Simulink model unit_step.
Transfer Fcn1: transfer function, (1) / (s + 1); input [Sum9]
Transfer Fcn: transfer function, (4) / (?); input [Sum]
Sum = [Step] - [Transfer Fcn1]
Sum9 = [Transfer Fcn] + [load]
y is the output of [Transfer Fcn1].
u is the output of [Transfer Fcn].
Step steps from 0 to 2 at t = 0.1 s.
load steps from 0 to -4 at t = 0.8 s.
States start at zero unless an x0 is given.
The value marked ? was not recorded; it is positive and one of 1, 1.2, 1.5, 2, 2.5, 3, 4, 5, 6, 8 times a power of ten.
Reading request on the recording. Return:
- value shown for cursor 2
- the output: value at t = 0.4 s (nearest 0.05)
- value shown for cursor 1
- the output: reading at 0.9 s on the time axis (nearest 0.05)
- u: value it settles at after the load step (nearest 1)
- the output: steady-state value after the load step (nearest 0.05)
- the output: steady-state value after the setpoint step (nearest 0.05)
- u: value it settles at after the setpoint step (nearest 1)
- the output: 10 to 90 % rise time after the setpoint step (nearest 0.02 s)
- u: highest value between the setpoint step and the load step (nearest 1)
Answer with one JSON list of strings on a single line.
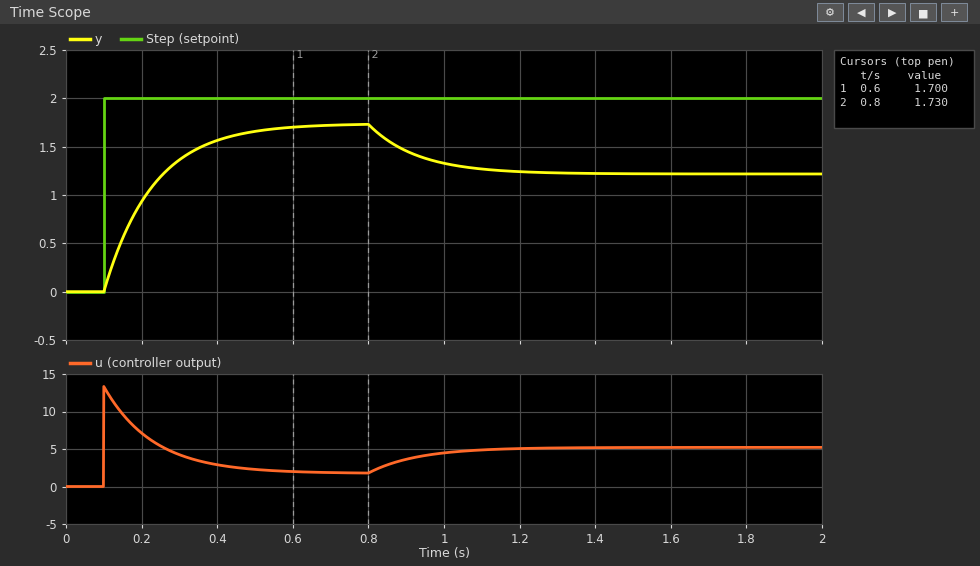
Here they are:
["1.730", "1.55", "1.700", "1.45", "5", "1.20", "1.75", "2", "0.28 s", "13"]
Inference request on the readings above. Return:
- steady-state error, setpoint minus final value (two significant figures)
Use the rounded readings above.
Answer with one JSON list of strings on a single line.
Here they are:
["0.25"]
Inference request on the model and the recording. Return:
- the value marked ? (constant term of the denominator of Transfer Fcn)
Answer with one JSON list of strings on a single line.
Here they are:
["0.6"]
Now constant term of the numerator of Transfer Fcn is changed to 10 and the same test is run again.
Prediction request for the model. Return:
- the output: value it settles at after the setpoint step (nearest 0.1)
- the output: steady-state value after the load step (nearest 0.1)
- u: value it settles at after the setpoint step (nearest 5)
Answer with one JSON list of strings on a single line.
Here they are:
["1.9", "1.7", "0"]
